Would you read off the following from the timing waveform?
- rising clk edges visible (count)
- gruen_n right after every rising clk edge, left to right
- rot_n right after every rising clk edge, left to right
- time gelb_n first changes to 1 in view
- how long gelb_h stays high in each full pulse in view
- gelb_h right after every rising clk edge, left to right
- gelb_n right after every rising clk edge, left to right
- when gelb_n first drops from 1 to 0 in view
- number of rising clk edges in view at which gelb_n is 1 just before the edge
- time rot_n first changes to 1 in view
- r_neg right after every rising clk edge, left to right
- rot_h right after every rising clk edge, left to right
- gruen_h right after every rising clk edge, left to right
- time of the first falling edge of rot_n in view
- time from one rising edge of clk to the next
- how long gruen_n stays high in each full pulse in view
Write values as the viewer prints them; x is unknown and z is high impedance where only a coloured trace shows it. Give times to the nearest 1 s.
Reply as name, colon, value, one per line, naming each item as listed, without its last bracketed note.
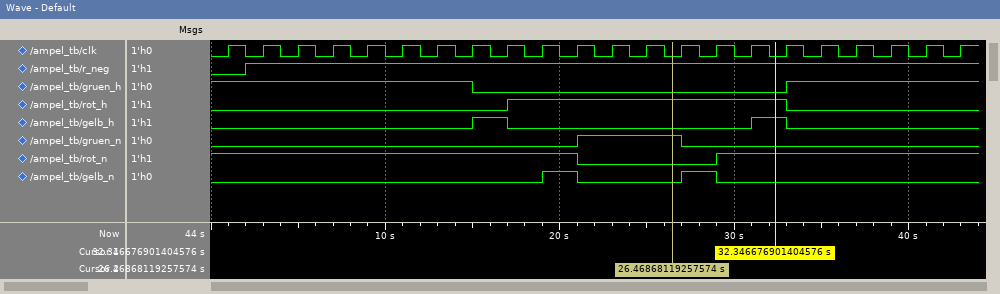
rising clk edges visible: 22
gruen_n right after every rising clk edge, left to right: 0 0 0 0 0 0 0 0 0 0 1 1 1 0 0 0 0 0 0 0 0 0
rot_n right after every rising clk edge, left to right: 1 1 1 1 1 1 1 1 1 1 0 0 0 0 1 1 1 1 1 1 1 1
time gelb_n first changes to 1 in view: 19 s
how long gelb_h stays high in each full pulse in view: 2 s, 2 s
gelb_h right after every rising clk edge, left to right: 0 0 0 0 0 0 0 1 0 0 0 0 0 0 0 1 0 0 0 0 0 0
gelb_n right after every rising clk edge, left to right: 0 0 0 0 0 0 0 0 0 1 0 0 0 1 0 0 0 0 0 0 0 0
when gelb_n first drops from 1 to 0 in view: 21 s
number of rising clk edges in view at which gelb_n is 1 just before the edge: 2
time rot_n first changes to 1 in view: 29 s
r_neg right after every rising clk edge, left to right: 0 1 1 1 1 1 1 1 1 1 1 1 1 1 1 1 1 1 1 1 1 1
rot_h right after every rising clk edge, left to right: 0 0 0 0 0 0 0 0 1 1 1 1 1 1 1 1 0 0 0 0 0 0
gruen_h right after every rising clk edge, left to right: 1 1 1 1 1 1 1 0 0 0 0 0 0 0 0 0 1 1 1 1 1 1
time of the first falling edge of rot_n in view: 21 s
time from one rising edge of clk to the next: 2 s
how long gruen_n stays high in each full pulse in view: 6 s
